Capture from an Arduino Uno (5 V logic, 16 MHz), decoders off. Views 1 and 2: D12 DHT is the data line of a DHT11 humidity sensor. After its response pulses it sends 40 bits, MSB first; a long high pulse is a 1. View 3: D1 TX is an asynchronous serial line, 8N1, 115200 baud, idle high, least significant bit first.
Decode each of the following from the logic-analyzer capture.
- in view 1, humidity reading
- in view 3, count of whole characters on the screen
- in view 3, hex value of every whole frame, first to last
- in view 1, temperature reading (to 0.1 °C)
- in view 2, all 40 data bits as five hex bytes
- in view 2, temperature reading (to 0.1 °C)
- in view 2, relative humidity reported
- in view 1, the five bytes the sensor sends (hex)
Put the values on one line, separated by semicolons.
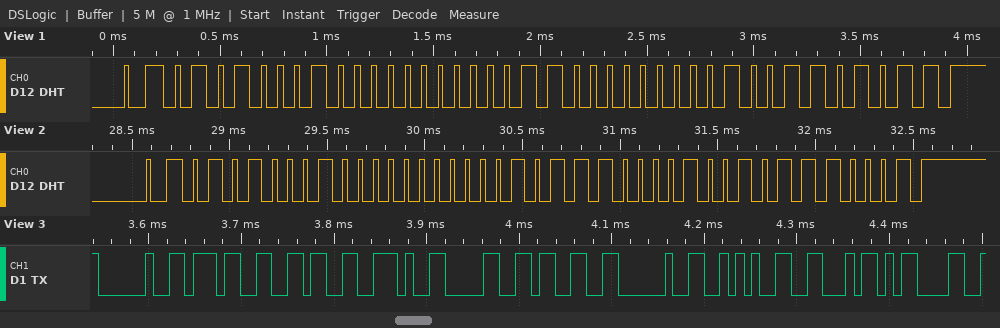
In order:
81 %; 10; 0x20 0x37 0x36 0x2E 0x30 0x33 0x20 0x2A 0x46 0x0D; 24.2 °C; 51 00 17 09 71; 23.9 °C; 81 %; 51 00 18 02 6B
